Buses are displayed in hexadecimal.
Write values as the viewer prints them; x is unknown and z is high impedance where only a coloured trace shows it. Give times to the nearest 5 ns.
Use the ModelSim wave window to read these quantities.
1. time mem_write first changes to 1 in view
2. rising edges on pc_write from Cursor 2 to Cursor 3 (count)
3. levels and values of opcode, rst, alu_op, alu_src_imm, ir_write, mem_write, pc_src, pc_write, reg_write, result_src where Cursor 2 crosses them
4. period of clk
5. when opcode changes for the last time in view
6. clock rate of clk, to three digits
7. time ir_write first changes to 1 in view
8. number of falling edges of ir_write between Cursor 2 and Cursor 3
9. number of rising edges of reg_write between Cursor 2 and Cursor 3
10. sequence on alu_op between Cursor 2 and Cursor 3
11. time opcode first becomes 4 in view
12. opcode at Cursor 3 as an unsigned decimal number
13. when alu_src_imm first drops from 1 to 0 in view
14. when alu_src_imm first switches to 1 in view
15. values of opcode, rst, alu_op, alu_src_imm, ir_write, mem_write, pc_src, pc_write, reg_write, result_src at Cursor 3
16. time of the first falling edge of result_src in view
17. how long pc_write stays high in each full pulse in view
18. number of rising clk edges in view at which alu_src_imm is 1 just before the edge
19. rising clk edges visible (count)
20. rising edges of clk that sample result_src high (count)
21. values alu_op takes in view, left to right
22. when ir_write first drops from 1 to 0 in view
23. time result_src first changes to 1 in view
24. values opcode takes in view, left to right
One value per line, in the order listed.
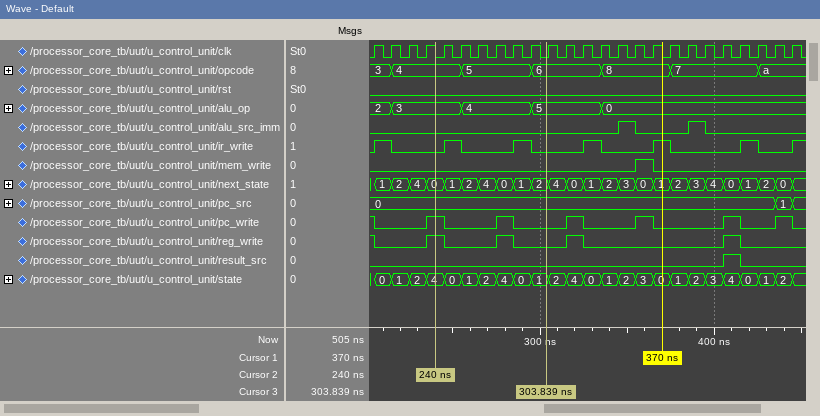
355 ns
1
opcode=4, rst=0, alu_op=3, alu_src_imm=0, ir_write=0, mem_write=0, pc_src=0, pc_write=1, reg_write=1, result_src=0
10 ns
425 ns
100 MHz
205 ns
2
1
3, 4, 5
215 ns
6
355 ns
345 ns
opcode=6, rst=0, alu_op=5, alu_src_imm=0, ir_write=0, mem_write=0, pc_src=0, pc_write=0, reg_write=0, result_src=0
415 ns
10 ns, 10 ns, 10 ns, 10 ns, 10 ns, 10 ns
2
25
1
2, 3, 4, 5, 0
215 ns
405 ns
3, 4, 5, 6, 8, 7, a
